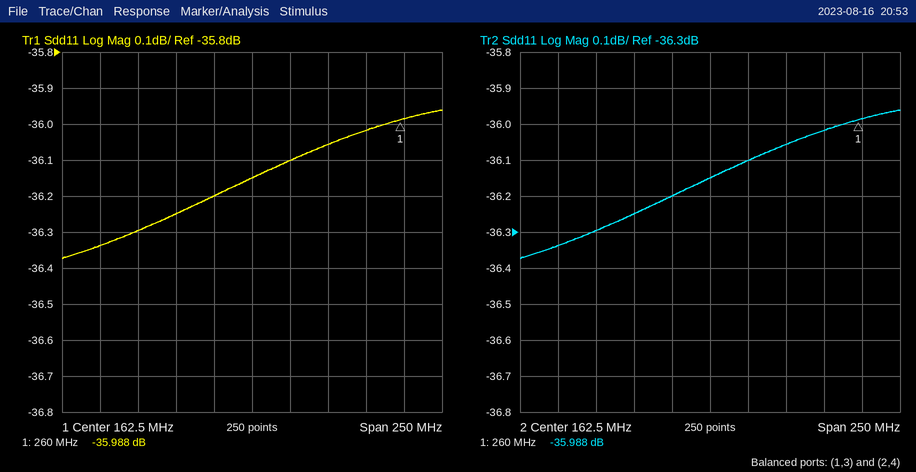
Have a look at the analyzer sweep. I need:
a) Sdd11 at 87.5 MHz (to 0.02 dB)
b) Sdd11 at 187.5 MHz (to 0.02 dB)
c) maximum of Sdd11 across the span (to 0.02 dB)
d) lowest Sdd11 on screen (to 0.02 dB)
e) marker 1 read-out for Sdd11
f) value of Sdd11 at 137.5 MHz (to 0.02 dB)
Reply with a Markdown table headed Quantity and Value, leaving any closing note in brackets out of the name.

| Quantity | Value |
|---|---|
| Sdd11 at 87.5 MHz | -36.30 dB |
| Sdd11 at 187.5 MHz | -36.10 dB |
| maximum of Sdd11 across the span | -35.96 dB |
| lowest Sdd11 on screen | -36.38 dB |
| marker 1 read-out for Sdd11 | -35.988 dB |
| value of Sdd11 at 137.5 MHz | -36.20 dB |
